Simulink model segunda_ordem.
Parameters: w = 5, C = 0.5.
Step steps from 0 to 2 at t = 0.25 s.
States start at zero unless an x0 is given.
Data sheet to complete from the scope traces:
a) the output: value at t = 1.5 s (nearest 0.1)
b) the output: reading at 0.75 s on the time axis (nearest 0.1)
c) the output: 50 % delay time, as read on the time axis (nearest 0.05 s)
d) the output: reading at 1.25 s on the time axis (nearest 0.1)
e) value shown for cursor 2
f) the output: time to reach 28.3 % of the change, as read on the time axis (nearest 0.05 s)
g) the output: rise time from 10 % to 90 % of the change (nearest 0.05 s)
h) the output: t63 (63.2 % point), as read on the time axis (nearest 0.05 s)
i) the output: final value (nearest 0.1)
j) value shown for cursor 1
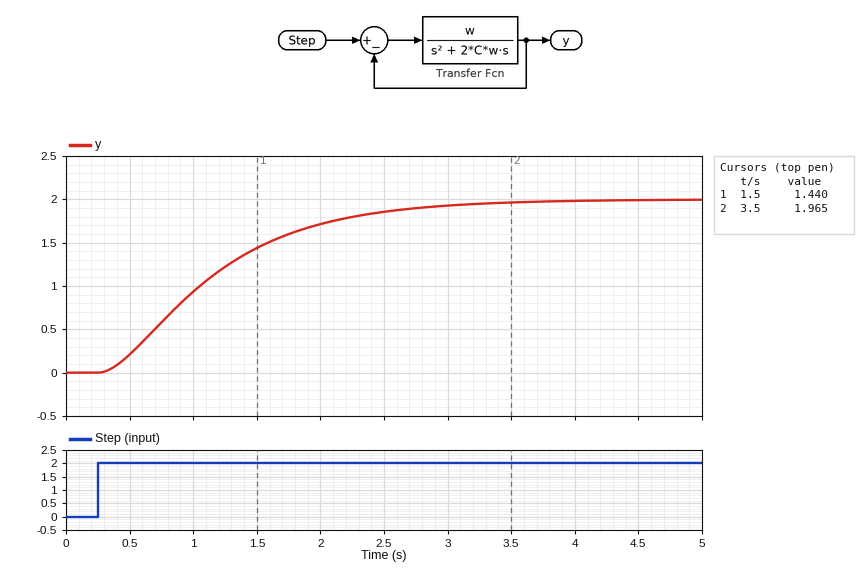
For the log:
1.4
0.6
1.05 s
1.2
1.965
0.75 s
1.75 s
1.30 s
2.0
1.440
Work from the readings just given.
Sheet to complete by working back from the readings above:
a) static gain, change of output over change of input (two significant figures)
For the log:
1.0
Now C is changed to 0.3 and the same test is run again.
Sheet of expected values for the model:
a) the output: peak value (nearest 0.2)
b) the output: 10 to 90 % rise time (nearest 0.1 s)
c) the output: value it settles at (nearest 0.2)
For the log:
2.2
0.9 s
2.0
